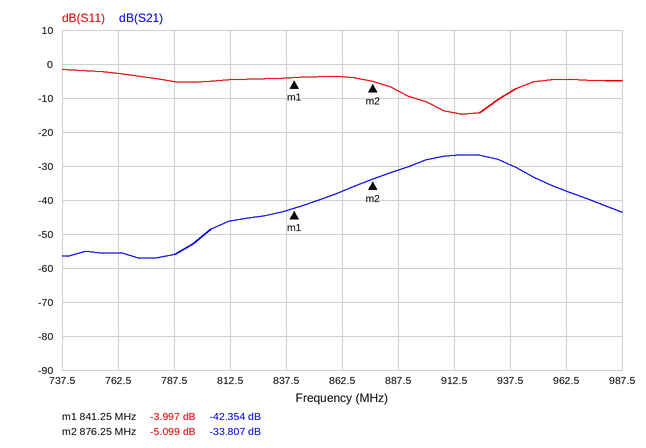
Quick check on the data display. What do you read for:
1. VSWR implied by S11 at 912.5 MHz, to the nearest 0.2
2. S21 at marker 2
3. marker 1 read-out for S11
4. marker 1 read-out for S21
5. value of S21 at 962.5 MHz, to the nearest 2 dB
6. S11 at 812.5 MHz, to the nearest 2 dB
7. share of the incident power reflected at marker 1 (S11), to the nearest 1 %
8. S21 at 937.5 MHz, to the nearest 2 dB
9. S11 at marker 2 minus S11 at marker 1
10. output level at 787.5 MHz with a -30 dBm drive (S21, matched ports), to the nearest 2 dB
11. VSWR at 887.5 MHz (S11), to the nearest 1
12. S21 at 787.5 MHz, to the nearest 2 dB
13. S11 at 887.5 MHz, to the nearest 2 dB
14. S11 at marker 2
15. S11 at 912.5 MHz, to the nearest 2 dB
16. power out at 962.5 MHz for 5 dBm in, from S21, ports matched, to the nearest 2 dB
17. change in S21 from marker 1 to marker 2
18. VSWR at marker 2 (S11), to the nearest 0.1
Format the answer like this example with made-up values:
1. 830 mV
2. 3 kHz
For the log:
1. 1.4
2. -33.807 dB
3. -3.997 dB
4. -42.354 dB
5. -38 dB
6. -4 dB
7. 40 %
8. -30 dB
9. -1.102 dB
10. -86 dBm
11. 2
12. -56 dB
13. -8 dB
14. -5.099 dB
15. -14 dB
16. -32 dBm
17. 8.547 dB
18. 3.5
